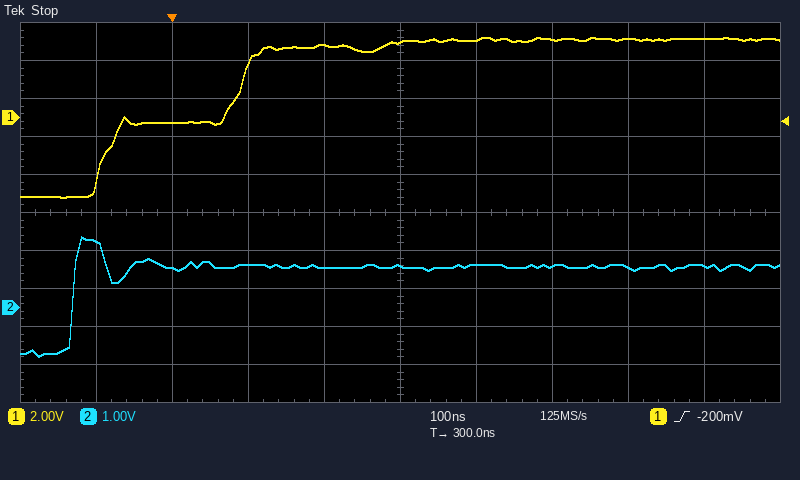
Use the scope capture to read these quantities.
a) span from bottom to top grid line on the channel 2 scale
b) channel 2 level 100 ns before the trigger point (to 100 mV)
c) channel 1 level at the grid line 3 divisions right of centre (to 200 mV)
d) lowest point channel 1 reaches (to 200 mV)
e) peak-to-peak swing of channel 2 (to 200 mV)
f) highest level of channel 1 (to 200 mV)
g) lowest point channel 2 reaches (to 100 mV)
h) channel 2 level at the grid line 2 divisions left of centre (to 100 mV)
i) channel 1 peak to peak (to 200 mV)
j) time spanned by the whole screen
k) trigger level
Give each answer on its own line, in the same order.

10 V
1.7 V
4.2 V
-4.2 V
3.2 V
4.2 V
-1.3 V
1.1 V
8.4 V
1 µs
-200 mV
